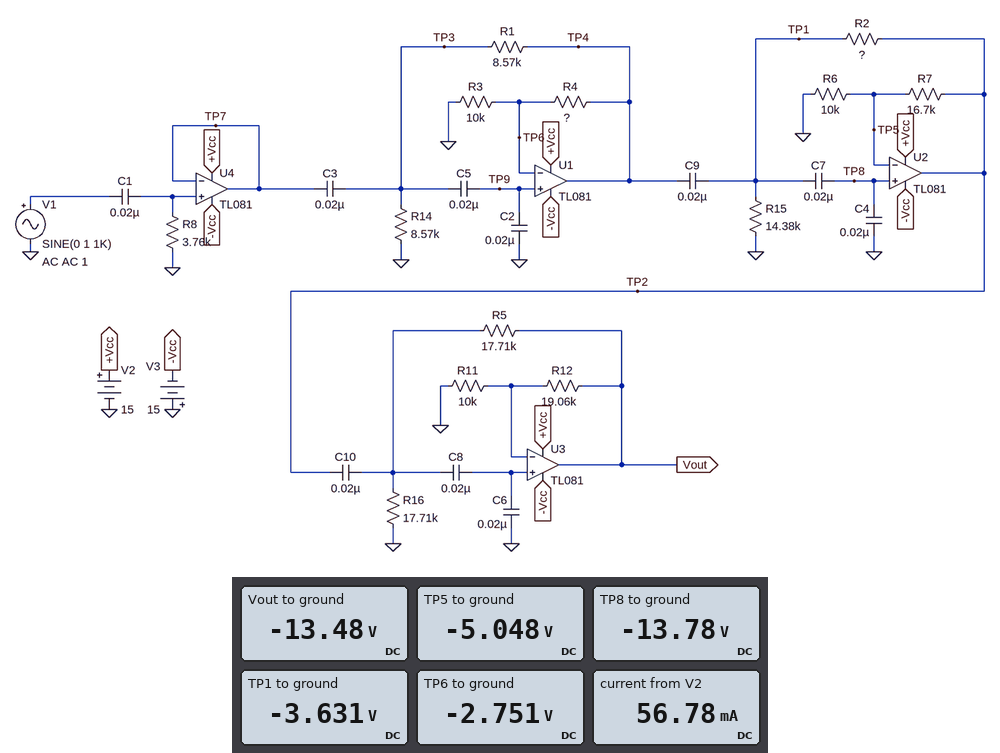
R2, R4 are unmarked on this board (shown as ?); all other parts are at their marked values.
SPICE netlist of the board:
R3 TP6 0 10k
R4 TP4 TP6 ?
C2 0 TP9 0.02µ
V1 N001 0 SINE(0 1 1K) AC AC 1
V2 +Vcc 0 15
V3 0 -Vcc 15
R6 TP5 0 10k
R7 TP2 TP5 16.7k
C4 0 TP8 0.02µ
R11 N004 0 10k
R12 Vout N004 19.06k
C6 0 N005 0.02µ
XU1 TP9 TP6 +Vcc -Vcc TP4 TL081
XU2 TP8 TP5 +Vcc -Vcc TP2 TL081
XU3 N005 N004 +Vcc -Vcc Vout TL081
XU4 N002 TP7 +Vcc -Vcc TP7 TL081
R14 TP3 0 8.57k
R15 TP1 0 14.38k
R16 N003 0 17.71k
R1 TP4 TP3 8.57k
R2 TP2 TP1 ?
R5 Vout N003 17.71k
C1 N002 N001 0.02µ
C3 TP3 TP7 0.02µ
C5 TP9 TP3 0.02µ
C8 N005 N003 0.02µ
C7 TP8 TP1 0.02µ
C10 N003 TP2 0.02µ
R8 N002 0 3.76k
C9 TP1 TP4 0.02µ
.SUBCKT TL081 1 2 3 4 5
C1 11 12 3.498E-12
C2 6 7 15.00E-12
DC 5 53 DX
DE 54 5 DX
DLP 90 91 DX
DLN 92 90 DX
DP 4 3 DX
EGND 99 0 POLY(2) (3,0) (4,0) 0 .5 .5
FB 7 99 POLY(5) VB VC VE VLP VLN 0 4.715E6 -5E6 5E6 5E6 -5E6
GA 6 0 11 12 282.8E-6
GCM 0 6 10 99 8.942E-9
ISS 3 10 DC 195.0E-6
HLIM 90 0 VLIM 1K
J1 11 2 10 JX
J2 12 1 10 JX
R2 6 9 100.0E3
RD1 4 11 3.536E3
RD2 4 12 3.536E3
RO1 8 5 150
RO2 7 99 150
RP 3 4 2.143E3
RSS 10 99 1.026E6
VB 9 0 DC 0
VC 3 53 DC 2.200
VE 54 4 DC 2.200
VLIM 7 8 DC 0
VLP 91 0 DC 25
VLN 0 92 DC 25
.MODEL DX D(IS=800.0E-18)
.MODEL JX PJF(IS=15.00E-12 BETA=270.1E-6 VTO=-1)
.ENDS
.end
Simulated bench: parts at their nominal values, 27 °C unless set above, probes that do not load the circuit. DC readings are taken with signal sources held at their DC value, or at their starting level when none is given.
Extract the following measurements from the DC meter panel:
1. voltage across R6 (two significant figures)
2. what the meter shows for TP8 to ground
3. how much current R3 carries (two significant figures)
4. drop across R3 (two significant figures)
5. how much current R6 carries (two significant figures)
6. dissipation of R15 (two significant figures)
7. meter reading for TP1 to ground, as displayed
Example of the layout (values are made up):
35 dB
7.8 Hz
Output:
5.0 V
-13.78 V
280 µA
2.8 V
500 µA
920 µW
-3.631 V
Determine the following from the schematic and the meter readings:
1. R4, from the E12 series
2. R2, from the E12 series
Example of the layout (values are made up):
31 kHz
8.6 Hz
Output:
39 kΩ
39 kΩ
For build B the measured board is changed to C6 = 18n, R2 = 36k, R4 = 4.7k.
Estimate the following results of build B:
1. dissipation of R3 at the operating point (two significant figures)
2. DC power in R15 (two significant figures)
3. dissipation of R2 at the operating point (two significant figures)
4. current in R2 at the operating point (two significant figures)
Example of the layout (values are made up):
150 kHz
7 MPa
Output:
8.4 mW
1.0 mW
2.6 mW
270 µA
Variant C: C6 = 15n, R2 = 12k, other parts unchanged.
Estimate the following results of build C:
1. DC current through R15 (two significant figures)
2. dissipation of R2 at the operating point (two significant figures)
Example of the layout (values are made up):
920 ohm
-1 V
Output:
510 µA
3.1 mW
